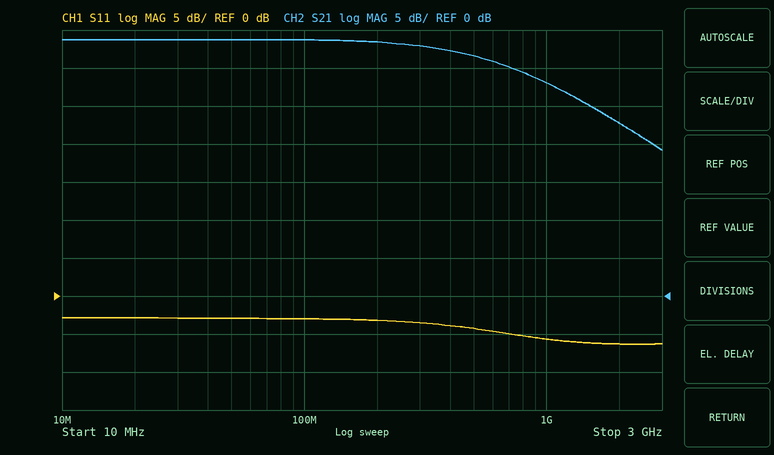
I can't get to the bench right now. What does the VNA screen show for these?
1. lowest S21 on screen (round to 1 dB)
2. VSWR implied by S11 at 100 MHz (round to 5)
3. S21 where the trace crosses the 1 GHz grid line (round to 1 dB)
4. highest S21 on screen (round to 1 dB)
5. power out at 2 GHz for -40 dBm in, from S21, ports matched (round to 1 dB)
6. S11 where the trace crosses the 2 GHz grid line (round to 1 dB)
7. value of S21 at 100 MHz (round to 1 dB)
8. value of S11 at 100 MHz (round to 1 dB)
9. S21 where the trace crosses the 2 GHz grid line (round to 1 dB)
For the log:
19 dB
5
28 dB
34 dB
-17 dBm
-6 dB
34 dB
-3 dB
23 dB
